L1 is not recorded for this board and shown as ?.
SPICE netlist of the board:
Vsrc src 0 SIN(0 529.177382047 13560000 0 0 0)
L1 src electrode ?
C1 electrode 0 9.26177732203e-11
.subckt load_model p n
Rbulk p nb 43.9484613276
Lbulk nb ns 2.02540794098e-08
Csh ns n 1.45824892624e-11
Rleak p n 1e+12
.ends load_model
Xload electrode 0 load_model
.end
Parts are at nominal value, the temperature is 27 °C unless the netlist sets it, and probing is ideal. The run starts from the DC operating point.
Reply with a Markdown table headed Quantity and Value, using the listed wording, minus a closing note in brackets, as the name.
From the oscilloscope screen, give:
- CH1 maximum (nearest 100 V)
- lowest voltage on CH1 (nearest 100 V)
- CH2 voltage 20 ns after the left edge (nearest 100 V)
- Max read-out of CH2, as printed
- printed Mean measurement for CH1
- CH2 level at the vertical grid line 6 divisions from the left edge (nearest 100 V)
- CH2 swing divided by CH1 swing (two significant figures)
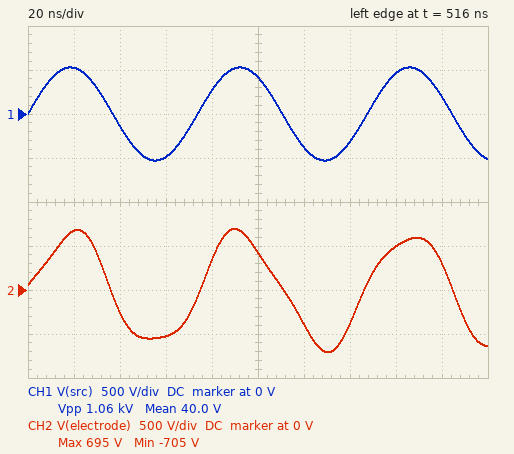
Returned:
| Quantity | Value |
|---|---|
| CH1 maximum | 500 V |
| lowest voltage on CH1 | -500 V |
| CH2 voltage 20 ns after the left edge | 700 V |
| Max read-out of CH2, as printed | 695 V |
| printed Mean measurement for CH1 | 40.0 V |
| CH2 level at the vertical grid line 6 divisions from the left edge | -400 V |
| CH2 swing divided by CH1 swing | 1.3 |
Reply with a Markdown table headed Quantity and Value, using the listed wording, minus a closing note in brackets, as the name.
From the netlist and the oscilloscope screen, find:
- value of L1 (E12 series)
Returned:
| Quantity | Value |
|---|---|
| value of L1 | 220 nH |
